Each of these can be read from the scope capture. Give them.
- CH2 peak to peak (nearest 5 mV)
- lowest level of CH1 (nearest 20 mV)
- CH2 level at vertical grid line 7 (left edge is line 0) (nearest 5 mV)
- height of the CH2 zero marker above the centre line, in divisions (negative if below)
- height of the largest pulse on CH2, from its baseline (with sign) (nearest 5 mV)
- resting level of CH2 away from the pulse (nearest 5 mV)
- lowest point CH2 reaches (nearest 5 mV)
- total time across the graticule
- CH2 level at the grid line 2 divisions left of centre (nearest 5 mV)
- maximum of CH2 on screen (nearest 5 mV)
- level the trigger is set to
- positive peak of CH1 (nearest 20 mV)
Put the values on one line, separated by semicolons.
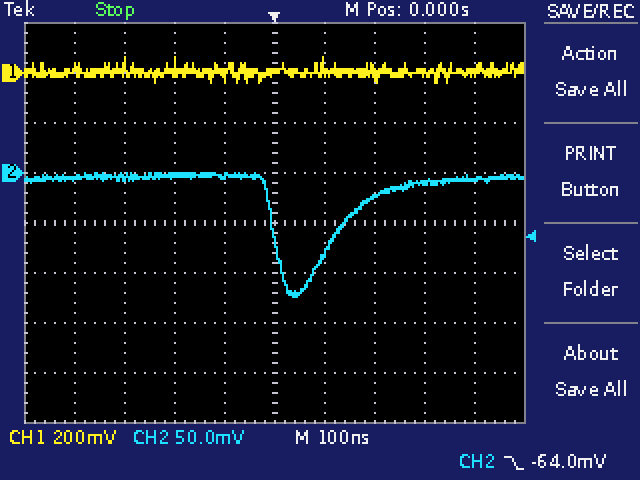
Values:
125 mV; -40 mV; -25 mV; +1.0 div; -120 mV; -5 mV; -125 mV; 1 µs; -5 mV; 0 mV; -64.0 mV; 60 mV
